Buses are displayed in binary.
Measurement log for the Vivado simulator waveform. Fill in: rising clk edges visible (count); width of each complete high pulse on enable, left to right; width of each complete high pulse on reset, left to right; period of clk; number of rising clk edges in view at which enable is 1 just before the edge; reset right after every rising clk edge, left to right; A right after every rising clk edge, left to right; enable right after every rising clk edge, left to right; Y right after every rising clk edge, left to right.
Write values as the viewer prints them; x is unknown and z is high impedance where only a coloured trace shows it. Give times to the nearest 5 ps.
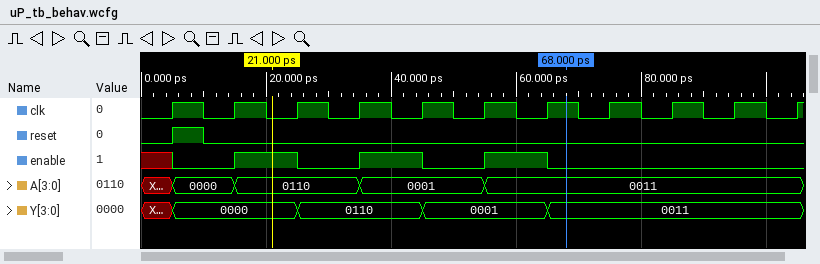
11
10 ps, 10 ps, 10 ps
5 ps
10 ps
3
1 0 0 0 0 0 0 0 0 0 0
0000, 0110, 0110, 0001, 0001, 0011, 0011, 0011, 0011, 0011, 0011
0 1 0 1 0 1 0 0 0 0 0
0000, 0000, 0110, 0110, 0001, 0001, 0011, 0011, 0011, 0011, 0011
